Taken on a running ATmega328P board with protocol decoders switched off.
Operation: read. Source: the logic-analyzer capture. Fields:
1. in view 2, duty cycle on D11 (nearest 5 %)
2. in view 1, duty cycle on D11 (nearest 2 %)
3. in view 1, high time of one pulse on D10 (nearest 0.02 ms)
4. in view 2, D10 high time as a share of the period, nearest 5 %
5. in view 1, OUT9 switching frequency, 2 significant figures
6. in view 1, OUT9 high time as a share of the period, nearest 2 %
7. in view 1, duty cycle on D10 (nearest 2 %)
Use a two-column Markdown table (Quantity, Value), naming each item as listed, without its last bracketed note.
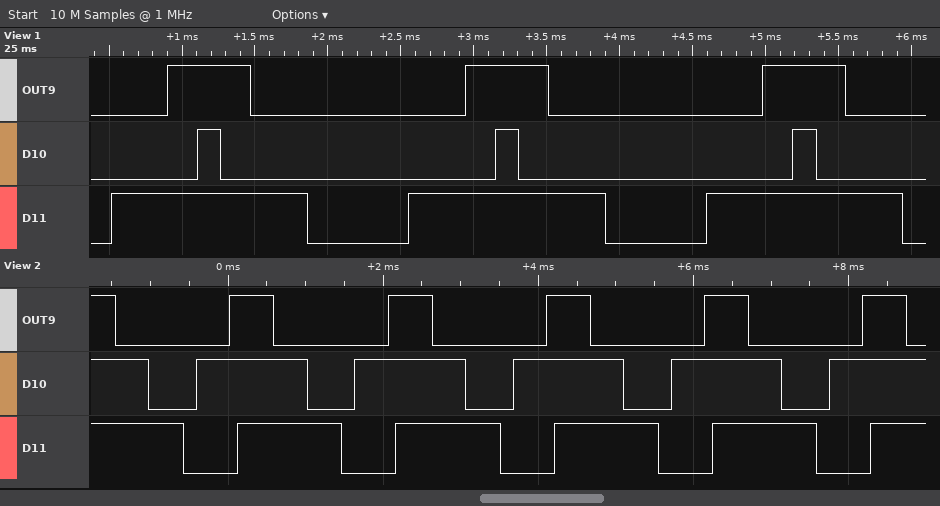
| Quantity | Value |
|---|---|
| in view 2, duty cycle on D11 | 65 % |
| in view 1, duty cycle on D11 | 66 % |
| in view 1, high time of one pulse on D10 | 0.16 ms |
| in view 2, D10 high time as a share of the period, nearest 5 % | 70 % |
| in view 1, OUT9 switching frequency, 2 significant figures | 490 Hz |
| in view 1, OUT9 high time as a share of the period, nearest 2 % | 28 % |
| in view 1, duty cycle on D10 | 8 % |
